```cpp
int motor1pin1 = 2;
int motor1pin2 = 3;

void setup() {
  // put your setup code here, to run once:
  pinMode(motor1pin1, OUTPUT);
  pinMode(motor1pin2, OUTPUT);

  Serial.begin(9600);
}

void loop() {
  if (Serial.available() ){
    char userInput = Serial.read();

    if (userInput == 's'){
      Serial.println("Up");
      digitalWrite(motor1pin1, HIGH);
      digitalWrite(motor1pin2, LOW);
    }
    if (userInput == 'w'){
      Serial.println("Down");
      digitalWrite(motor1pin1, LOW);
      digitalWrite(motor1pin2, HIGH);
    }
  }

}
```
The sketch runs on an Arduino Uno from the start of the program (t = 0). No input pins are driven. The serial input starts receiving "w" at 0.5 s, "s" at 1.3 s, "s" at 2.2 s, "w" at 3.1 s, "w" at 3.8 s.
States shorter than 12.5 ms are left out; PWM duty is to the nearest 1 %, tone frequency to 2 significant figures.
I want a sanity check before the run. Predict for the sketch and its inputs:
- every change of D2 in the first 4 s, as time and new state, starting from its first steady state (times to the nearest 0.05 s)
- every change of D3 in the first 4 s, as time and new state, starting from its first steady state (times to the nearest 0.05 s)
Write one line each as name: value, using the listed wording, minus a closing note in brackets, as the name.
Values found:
every change of D2 in the first 4 s, as time and new state, starting from its first steady state: 0 s low; 1.3 s high; 3.1 s low
every change of D3 in the first 4 s, as time and new state, starting from its first steady state: 0 s low; 0.5 s high; 1.3 s low; 3.1 s high
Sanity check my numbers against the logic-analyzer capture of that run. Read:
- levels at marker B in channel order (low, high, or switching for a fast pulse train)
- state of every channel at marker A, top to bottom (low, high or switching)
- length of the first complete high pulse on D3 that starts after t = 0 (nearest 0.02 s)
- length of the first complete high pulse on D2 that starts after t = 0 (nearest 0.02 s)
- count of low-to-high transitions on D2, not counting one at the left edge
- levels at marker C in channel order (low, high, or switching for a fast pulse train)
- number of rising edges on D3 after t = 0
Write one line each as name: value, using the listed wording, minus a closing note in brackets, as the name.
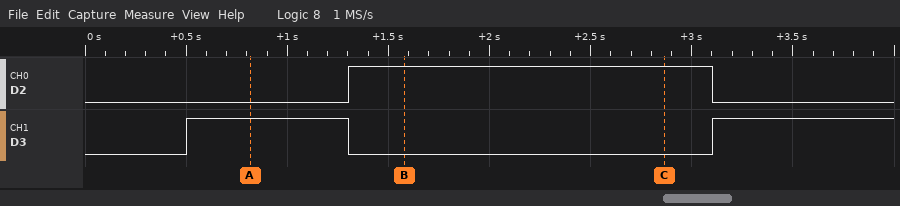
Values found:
levels at marker B in channel order: D2 high, D3 low
state of every channel at marker A, top to bottom: D2 low, D3 high
length of the first complete high pulse on D3 that starts after t = 0: 0.80 s
length of the first complete high pulse on D2 that starts after t = 0: 1.80 s
count of low-to-high transitions on D2, not counting one at the left edge: 1
levels at marker C in channel order: D2 high, D3 low
number of rising edges on D3 after t = 0: 2
